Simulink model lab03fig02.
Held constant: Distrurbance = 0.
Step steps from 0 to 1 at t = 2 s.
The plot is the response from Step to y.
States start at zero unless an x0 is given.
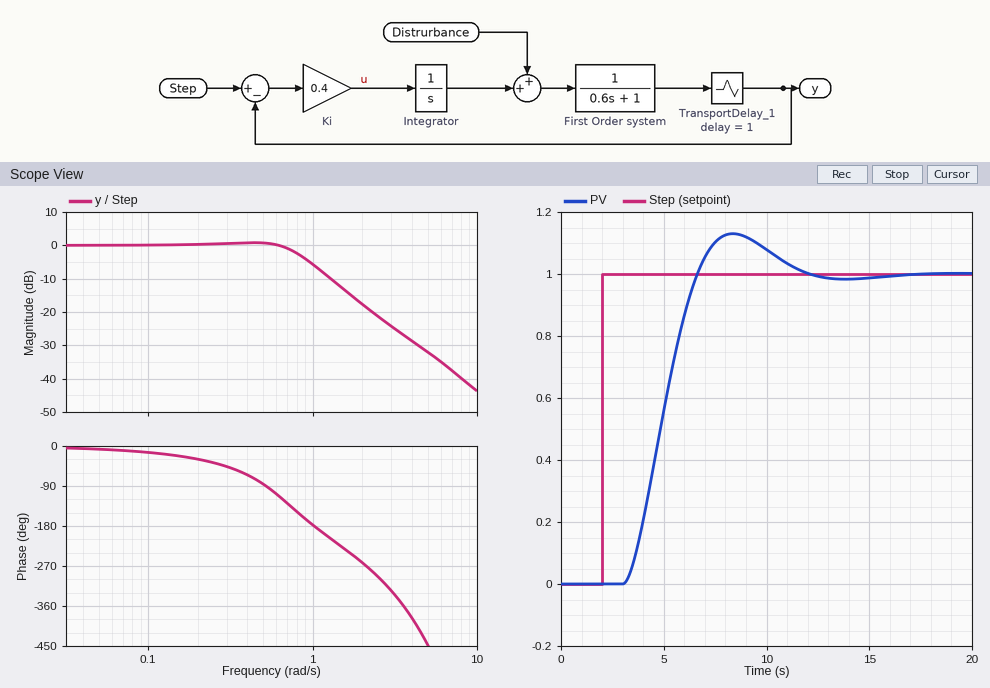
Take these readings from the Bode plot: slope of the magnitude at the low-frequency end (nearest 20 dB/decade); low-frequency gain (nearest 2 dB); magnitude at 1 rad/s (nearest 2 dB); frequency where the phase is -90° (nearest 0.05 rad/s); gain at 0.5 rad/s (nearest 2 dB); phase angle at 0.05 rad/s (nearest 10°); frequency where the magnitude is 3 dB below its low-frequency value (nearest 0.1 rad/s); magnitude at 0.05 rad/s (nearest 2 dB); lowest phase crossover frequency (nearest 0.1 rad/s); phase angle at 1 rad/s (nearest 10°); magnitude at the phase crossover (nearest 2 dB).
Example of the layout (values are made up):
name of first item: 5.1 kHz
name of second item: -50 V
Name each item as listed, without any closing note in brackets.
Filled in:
slope of the magnitude at the low-frequency end: 0 dB/decade
low-frequency gain: 0 dB
magnitude at 1 rad/s: -6 dB
frequency where the phase is -90°: 0.50 rad/s
gain at 0.5 rad/s: 0 dB
phase angle at 0.05 rad/s: -10°
frequency where the magnitude is 3 dB below its low-frequency value: 0.8 rad/s
magnitude at 0.05 rad/s: 0 dB
lowest phase crossover frequency: 1.0 rad/s
phase angle at 1 rad/s: -180°
magnitude at the phase crossover: -6 dB
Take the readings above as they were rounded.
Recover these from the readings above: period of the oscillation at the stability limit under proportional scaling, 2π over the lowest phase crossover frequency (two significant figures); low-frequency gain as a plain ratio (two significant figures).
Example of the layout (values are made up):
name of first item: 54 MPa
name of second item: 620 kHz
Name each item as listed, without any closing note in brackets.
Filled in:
period of the oscillation at the stability limit under proportional scaling, 2π over the lowest phase crossover frequency: 6.3 s
low-frequency gain as a plain ratio: 1.0
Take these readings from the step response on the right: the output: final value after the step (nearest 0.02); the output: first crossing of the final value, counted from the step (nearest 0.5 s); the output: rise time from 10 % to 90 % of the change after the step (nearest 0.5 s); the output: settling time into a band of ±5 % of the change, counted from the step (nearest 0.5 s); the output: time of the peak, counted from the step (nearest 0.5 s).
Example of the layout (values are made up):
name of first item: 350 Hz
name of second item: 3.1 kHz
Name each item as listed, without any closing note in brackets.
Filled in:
the output: final value after the step: 1.00
the output: first crossing of the final value, counted from the step: 4.5 s
the output: rise time from 10 % to 90 % of the change after the step: 2.5 s
the output: settling time into a band of ±5 % of the change, counted from the step: 8.5 s
the output: time of the peak, counted from the step: 6.5 s
